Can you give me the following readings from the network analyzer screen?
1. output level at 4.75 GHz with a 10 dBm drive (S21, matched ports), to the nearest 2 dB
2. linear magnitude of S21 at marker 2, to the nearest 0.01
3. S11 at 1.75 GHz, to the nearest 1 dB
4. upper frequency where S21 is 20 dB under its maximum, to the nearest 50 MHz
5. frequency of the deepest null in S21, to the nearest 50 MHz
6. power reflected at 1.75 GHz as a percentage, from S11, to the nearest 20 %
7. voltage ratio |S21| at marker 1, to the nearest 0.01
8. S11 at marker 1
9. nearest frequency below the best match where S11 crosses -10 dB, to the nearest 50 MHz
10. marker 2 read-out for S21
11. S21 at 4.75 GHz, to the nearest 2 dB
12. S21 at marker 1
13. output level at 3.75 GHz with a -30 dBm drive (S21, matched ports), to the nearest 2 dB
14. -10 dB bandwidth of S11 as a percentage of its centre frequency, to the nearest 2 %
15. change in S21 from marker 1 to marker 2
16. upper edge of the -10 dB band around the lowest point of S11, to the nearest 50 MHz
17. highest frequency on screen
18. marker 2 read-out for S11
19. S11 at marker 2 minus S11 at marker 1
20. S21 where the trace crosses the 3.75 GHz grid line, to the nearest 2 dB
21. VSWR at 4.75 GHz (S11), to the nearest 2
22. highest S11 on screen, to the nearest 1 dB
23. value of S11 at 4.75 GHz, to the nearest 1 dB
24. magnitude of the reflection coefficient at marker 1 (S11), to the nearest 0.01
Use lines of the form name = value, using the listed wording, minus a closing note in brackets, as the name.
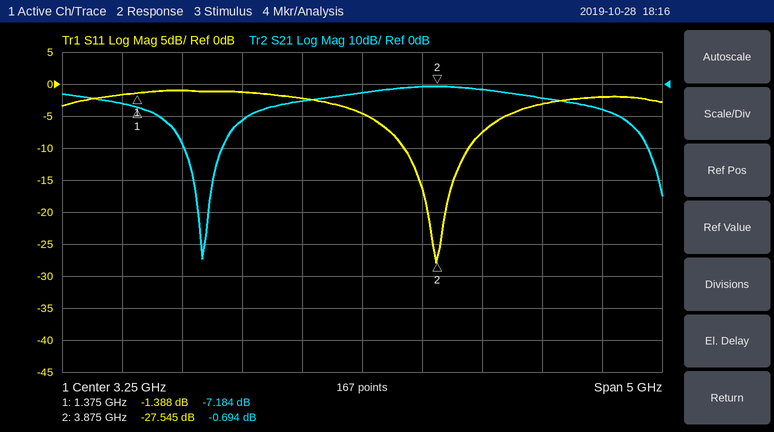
output level at 4.75 GHz with a 10 dBm drive (S21, matched ports), to the nearest 2 dB = 6 dBm
linear magnitude of S21 at marker 2, to the nearest 0.01 = 0.92
S11 at 1.75 GHz, to the nearest 1 dB = -1 dB
upper frequency where S21 is 20 dB under its maximum, to the nearest 50 MHz = 5.65 GHz
frequency of the deepest null in S21, to the nearest 50 MHz = 1.90 GHz
power reflected at 1.75 GHz as a percentage, from S11, to the nearest 20 % = 80 %
voltage ratio |S21| at marker 1, to the nearest 0.01 = 0.44
S11 at marker 1 = -1.388 dB
nearest frequency below the best match where S11 crosses -10 dB, to the nearest 50 MHz = 3.60 GHz
marker 2 read-out for S21 = -0.694 dB
S21 at 4.75 GHz, to the nearest 2 dB = -4 dB
S21 at marker 1 = -7.184 dB
output level at 3.75 GHz with a -30 dBm drive (S21, matched ports), to the nearest 2 dB = -30 dBm
-10 dB bandwidth of S11 as a percentage of its centre frequency, to the nearest 2 % = 14 %
change in S21 from marker 1 to marker 2 = 6.490 dB
upper edge of the -10 dB band around the lowest point of S11, to the nearest 50 MHz = 4.15 GHz
highest frequency on screen = 5.75 GHz
marker 2 read-out for S11 = -27.545 dB
S11 at marker 2 minus S11 at marker 1 = -26.157 dB
S21 where the trace crosses the 3.75 GHz grid line, to the nearest 2 dB = 0 dB
VSWR at 4.75 GHz (S11), to the nearest 2 = 6
highest S11 on screen, to the nearest 1 dB = -1 dB
value of S11 at 4.75 GHz, to the nearest 1 dB = -3 dB
magnitude of the reflection coefficient at marker 1 (S11), to the nearest 0.01 = 0.85
